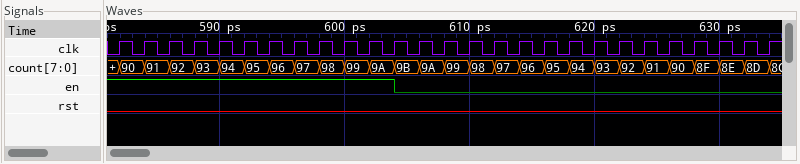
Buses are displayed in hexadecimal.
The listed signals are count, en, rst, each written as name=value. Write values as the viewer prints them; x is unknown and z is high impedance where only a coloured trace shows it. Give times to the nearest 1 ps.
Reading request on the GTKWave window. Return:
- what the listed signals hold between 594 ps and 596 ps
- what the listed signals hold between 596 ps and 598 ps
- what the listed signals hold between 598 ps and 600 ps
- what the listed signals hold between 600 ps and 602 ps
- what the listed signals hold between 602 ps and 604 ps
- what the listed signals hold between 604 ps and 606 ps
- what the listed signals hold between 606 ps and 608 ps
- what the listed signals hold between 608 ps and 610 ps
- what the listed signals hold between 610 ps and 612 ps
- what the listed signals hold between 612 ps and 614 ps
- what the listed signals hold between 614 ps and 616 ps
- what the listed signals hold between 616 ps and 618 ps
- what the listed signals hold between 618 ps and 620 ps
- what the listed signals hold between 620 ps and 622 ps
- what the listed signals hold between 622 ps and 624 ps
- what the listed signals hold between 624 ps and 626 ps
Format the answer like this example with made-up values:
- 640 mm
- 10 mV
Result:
- count=96, en=1, rst=0
- count=97, en=1, rst=0
- count=98, en=1, rst=0
- count=99, en=1, rst=0
- count=9A, en=1, rst=0
- count=9B, en=0, rst=0
- count=9A, en=0, rst=0
- count=99, en=0, rst=0
- count=98, en=0, rst=0
- count=97, en=0, rst=0
- count=96, en=0, rst=0
- count=95, en=0, rst=0
- count=94, en=0, rst=0
- count=93, en=0, rst=0
- count=92, en=0, rst=0
- count=91, en=0, rst=0
